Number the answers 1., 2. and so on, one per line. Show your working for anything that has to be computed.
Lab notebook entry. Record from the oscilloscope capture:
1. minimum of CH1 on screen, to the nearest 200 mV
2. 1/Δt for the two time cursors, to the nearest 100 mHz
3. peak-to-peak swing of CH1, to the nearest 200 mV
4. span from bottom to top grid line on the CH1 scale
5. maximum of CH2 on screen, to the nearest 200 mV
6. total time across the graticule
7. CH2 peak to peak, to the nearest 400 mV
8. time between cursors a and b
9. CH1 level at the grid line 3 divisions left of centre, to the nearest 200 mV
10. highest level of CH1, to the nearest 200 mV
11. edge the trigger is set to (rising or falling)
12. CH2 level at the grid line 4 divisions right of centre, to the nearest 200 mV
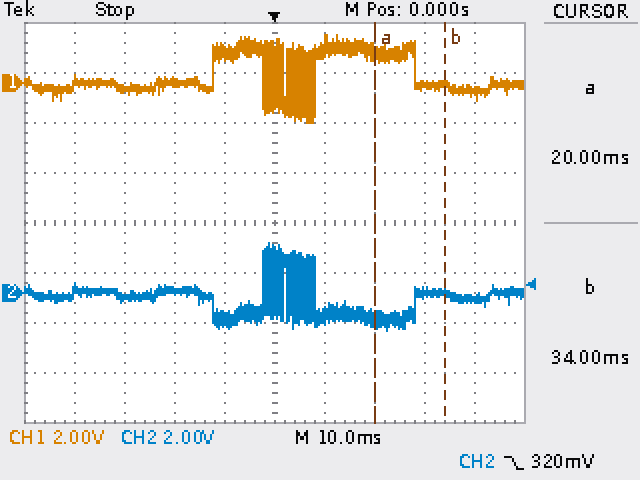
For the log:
1. -1.6 V
2. 1 / 14 ms ≈ 71.4 Hz
3. 2.0 V − (-1.6 V) = 3.6 V
4. 16 V
5. 2.0 V
6. 100 ms
7. 3.6 V
8. 34 ms − (20 ms) = 14 ms
9. -200 mV
10. 2.0 V
11. falling
12. -200 mV
